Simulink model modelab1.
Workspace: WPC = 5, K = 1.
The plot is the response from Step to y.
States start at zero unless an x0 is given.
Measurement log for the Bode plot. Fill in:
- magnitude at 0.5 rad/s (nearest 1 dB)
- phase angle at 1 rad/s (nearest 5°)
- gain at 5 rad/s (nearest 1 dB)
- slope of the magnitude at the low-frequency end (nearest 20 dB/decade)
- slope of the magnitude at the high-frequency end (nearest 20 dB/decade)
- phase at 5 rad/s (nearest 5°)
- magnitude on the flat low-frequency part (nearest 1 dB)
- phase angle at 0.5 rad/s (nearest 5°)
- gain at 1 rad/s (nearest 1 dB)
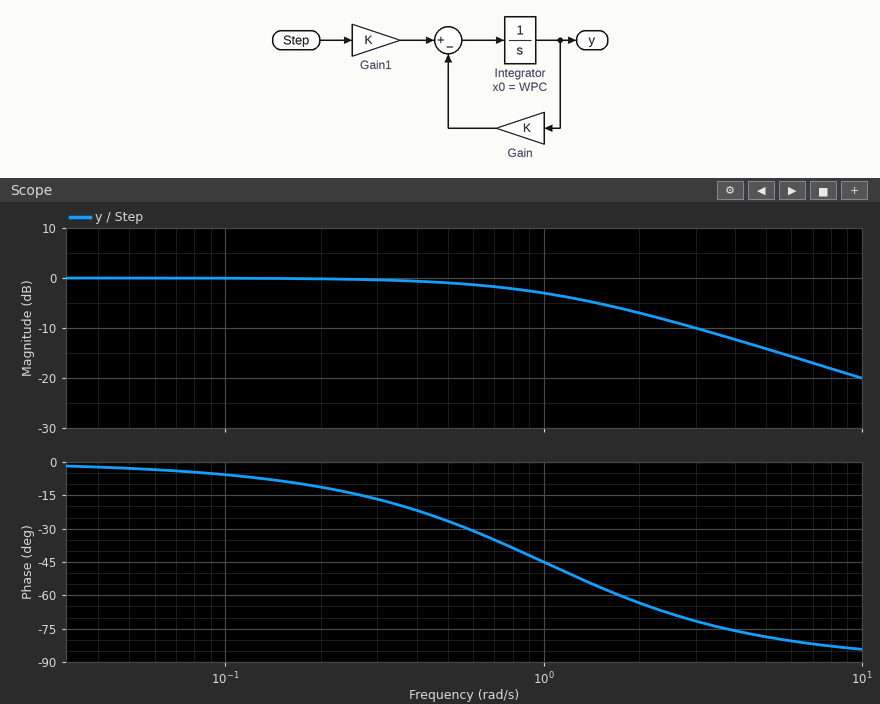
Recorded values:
-1 dB
-45°
-14 dB
0 dB/decade
-20 dB/decade
-80°
0 dB
-25°
-3 dB
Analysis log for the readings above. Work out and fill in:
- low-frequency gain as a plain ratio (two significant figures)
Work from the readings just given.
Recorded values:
1.0
